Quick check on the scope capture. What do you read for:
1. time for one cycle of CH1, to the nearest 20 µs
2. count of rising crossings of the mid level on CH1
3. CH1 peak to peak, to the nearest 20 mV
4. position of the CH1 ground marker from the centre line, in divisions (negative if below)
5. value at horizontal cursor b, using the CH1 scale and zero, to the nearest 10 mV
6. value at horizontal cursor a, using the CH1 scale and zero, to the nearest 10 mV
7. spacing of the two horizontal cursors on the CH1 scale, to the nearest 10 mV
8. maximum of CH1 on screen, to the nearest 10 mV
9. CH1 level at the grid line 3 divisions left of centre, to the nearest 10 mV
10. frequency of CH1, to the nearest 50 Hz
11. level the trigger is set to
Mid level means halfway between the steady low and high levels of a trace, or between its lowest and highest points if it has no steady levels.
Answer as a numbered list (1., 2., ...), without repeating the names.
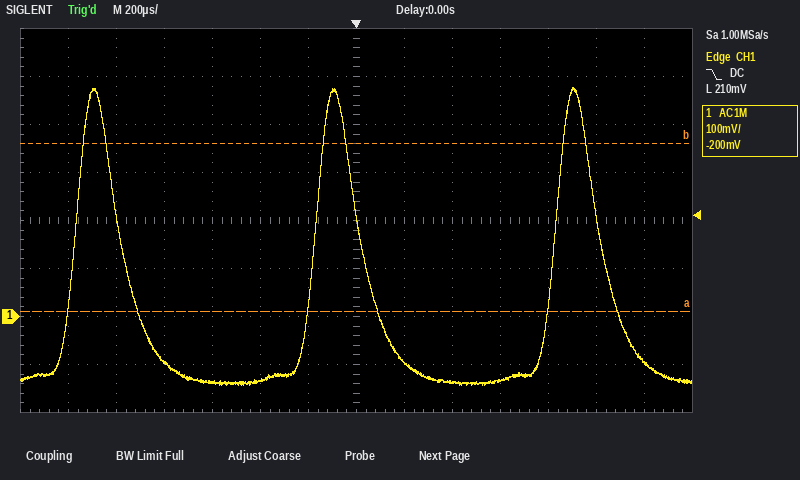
1. 1.00 ms
2. 3
3. 620 mV
4. -2.0 div
5. 360 mV
6. 10 mV
7. 350 mV
8. 480 mV
9. -140 mV
10. 1.00 kHz
11. 210 mV
